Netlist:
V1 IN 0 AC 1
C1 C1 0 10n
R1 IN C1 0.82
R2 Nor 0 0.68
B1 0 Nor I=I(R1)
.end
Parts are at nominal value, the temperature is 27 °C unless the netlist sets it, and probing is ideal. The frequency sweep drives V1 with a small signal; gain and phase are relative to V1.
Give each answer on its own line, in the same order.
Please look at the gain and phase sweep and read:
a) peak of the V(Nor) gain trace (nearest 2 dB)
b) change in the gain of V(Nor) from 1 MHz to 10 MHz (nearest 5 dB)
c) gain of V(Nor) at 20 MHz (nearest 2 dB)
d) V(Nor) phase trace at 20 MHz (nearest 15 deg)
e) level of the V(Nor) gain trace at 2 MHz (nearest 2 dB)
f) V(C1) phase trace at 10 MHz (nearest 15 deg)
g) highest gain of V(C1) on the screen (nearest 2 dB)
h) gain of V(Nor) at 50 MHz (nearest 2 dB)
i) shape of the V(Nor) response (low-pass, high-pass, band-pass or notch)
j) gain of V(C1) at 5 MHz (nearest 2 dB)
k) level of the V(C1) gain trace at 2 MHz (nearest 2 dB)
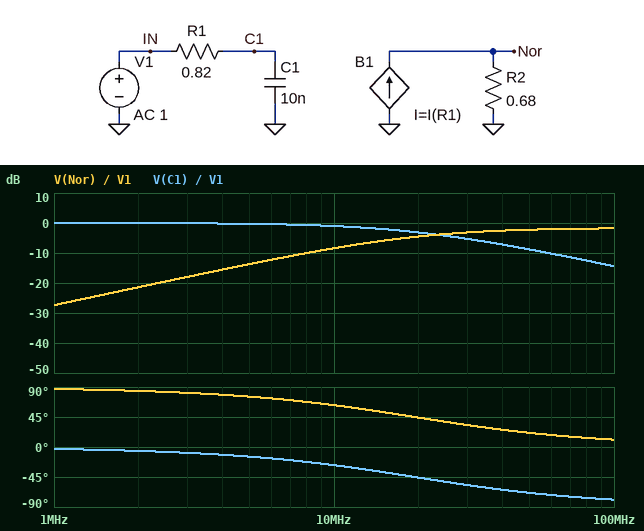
-2 dB
20 dB
-4 dB
45 deg
-22 dB
-30 deg
0 dB
-2 dB
high-pass
0 dB
0 dB
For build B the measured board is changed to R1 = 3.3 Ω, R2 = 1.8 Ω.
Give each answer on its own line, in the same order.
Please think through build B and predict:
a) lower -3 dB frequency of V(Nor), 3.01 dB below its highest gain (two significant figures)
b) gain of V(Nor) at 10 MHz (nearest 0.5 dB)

4.8 MHz
-6.0 dB
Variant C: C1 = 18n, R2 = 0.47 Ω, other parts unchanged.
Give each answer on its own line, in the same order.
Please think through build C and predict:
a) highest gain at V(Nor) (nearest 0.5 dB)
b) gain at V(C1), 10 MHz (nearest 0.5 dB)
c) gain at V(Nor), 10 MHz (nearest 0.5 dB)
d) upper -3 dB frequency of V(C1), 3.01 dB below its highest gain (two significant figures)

-5.0 dB
-2.5 dB
-8.0 dB
11 MHz
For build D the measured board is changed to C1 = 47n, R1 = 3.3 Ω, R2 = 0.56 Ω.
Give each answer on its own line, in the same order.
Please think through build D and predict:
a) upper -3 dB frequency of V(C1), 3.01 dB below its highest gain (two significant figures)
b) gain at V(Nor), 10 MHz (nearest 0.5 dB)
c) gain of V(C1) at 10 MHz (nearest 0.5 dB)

1.0 MHz
-15.5 dB
-20.0 dB
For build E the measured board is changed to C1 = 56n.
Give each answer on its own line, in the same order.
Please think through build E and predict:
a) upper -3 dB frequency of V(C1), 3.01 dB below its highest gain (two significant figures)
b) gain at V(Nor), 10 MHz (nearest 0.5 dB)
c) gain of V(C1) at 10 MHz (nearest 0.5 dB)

3.5 MHz
-2.0 dB
-9.5 dB
